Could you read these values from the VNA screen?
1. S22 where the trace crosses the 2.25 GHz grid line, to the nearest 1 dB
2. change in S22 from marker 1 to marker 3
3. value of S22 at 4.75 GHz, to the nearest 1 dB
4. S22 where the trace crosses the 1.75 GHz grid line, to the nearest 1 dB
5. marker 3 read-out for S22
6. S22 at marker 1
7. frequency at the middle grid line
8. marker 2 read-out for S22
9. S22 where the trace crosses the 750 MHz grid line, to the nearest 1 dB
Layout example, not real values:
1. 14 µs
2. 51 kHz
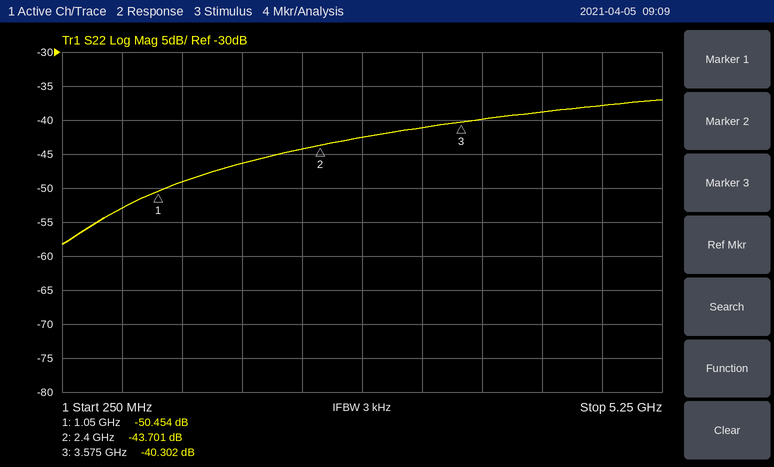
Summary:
1. -44 dB
2. 10.152 dB
3. -38 dB
4. -46 dB
5. -40.302 dB
6. -50.454 dB
7. 2.75 GHz
8. -43.701 dB
9. -53 dB
